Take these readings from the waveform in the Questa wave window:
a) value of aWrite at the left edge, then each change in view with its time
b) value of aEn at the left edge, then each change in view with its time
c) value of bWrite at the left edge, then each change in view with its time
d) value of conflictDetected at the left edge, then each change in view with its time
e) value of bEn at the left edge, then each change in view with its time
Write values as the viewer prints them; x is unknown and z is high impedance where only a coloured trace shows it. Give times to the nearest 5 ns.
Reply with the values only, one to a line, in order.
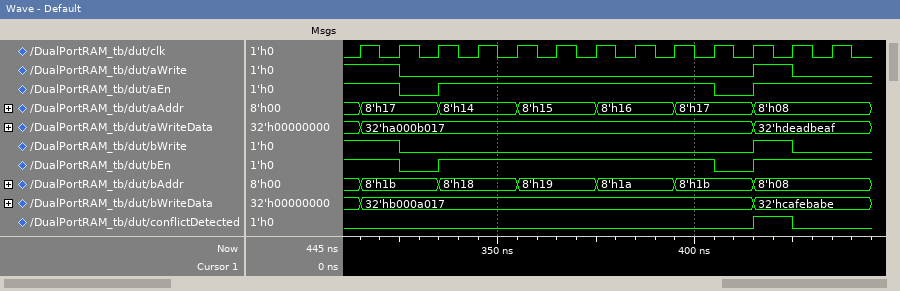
1, 0 at 325 ns, 1 at 415 ns, 0 at 425 ns
1, 0 at 325 ns, 1 at 335 ns, 0 at 405 ns, 1 at 415 ns
1, 0 at 325 ns, 1 at 415 ns, 0 at 425 ns
0, 1 at 415 ns, 0 at 425 ns
1, 0 at 325 ns, 1 at 335 ns, 0 at 405 ns, 1 at 415 ns
